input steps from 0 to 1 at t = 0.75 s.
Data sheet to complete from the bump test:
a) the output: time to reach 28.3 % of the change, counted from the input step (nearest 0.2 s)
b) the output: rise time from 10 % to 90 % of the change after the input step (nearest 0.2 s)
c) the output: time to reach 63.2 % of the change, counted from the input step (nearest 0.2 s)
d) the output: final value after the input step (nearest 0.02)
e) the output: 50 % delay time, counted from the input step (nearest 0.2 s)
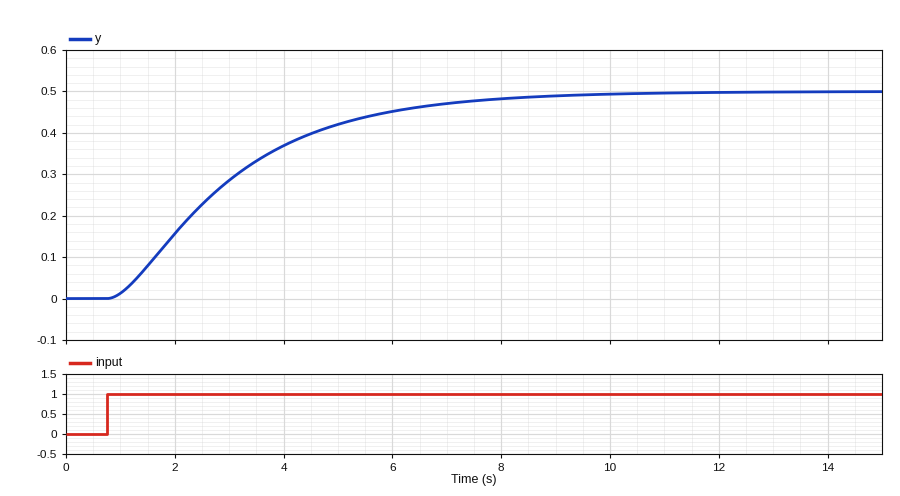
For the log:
1.2 s
4.6 s
2.6 s
0.50
2.0 s
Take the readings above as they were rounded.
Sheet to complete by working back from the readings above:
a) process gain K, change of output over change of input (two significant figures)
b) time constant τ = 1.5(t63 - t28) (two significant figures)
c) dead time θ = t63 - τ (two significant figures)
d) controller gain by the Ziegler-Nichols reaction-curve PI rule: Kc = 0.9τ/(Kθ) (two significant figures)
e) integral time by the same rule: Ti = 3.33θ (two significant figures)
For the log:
0.50
2.1 s
0.50 s
7.6
1.7 s
